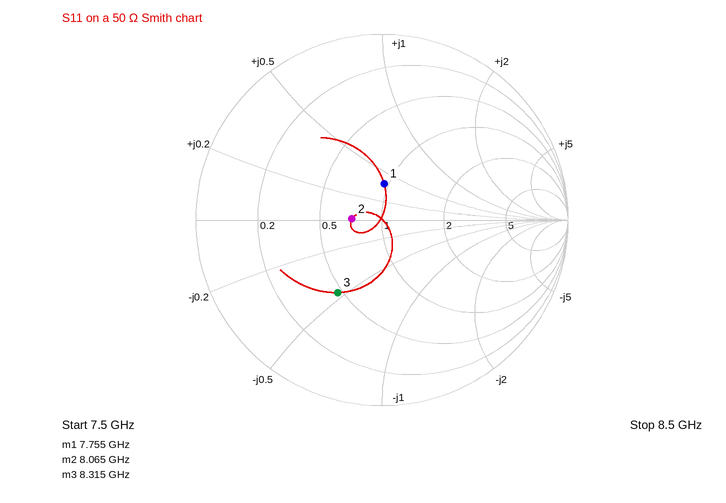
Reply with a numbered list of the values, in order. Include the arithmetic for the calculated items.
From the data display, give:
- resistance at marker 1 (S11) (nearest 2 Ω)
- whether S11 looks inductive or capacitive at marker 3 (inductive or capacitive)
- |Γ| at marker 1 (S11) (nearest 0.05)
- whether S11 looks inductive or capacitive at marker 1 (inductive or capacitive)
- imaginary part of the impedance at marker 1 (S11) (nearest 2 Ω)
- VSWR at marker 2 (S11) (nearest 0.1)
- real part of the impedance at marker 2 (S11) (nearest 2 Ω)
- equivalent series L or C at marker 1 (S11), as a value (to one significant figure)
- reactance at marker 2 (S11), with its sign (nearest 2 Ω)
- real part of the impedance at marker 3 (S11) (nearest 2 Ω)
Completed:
1. 48 Ω
2. capacitive
3. 0.20
4. inductive
5. +20 Ω
6. 1.4
7. 36 Ω
8. L = 20 Ω/(2π × 7.755 GHz) ≈ 410 pH, so 400 pH to one significant figure
9. 0 Ω
10. 24 Ω
